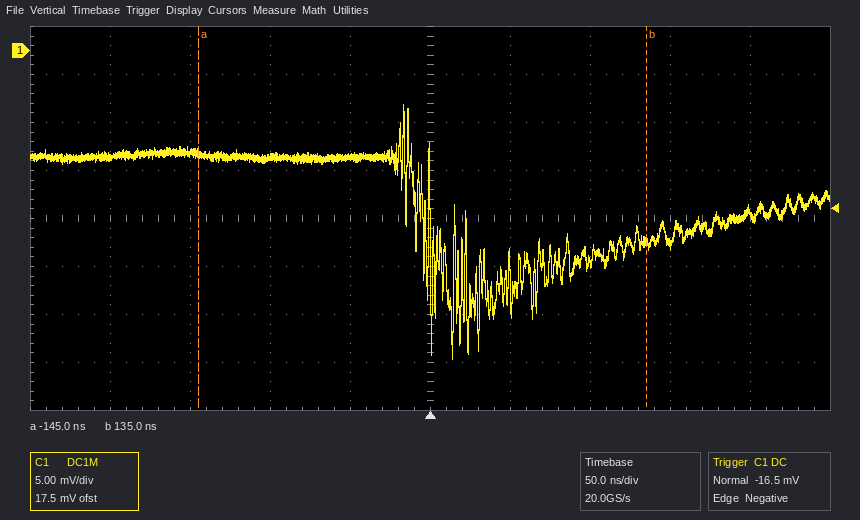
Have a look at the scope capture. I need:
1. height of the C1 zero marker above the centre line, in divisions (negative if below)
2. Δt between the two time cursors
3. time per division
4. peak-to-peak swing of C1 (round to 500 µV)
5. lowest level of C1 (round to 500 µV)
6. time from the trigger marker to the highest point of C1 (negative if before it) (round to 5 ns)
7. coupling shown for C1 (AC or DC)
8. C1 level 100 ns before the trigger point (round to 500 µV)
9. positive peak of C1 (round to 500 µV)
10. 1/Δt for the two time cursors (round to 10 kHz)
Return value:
+3.5 div
280 ns
50 ns
26.5 mV
-32.0 mV
-15 ns
DC
-11.0 mV
-5.5 mV
3.57 MHz
